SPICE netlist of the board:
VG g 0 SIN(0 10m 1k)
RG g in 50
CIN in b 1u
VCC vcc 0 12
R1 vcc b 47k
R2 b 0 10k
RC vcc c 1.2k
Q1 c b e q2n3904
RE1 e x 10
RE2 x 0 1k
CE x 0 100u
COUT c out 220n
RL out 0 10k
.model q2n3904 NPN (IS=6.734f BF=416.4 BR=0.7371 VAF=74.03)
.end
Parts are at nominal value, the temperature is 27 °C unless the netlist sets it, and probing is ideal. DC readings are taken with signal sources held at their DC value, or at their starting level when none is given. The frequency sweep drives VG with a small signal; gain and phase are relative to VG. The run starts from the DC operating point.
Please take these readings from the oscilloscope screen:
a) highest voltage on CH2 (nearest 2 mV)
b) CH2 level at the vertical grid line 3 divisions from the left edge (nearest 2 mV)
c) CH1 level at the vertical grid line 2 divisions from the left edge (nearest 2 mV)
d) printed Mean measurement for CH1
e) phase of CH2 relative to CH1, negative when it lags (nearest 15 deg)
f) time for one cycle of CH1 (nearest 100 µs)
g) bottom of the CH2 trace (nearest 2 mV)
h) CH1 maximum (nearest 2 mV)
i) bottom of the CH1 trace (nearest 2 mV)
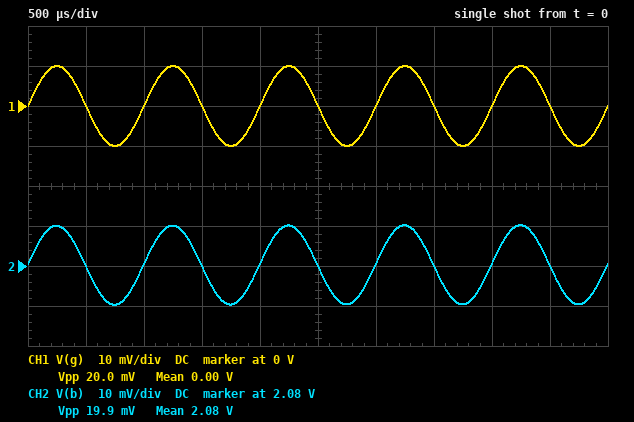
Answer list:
2.090 V
2.080 V
0 V
0.00 V
0 deg
1.0 ms
2.070 V
10 mV
-10 mV
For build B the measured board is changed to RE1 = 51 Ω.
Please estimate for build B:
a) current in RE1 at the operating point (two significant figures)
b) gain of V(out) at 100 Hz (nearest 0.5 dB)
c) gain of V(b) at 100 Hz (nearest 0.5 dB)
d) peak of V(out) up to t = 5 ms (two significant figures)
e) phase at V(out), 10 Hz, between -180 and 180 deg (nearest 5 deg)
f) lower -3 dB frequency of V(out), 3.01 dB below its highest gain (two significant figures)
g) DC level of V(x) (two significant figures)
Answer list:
1.3 mA
21.5 dB
-0.5 dB
160 mV
20 deg
81 Hz
1.3 V
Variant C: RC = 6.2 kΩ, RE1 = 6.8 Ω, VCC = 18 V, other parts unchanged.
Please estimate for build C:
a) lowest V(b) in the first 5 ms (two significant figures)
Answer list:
3.1 V
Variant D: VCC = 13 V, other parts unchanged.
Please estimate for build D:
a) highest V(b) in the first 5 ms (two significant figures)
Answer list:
2.3 V
